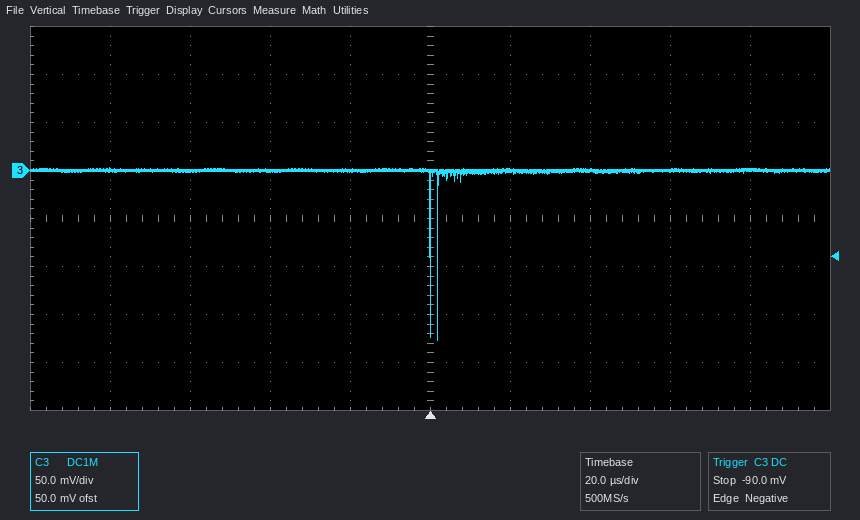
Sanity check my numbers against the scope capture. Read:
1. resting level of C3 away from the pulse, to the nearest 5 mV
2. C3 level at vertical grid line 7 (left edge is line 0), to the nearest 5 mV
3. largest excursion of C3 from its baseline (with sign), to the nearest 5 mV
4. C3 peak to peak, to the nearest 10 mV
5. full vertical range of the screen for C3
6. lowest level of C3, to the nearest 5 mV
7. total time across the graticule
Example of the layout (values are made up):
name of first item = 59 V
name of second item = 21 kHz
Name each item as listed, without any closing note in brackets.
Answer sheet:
resting level of C3 away from the pulse, to the nearest 5 mV = 0 mV
C3 level at vertical grid line 7 (left edge is line 0), to the nearest 5 mV = 0 mV
largest excursion of C3 from its baseline (with sign), to the nearest 5 mV = -175 mV
C3 peak to peak, to the nearest 10 mV = 180 mV
full vertical range of the screen for C3 = 400 mV
lowest level of C3, to the nearest 5 mV = -175 mV
total time across the graticule = 200 µs
